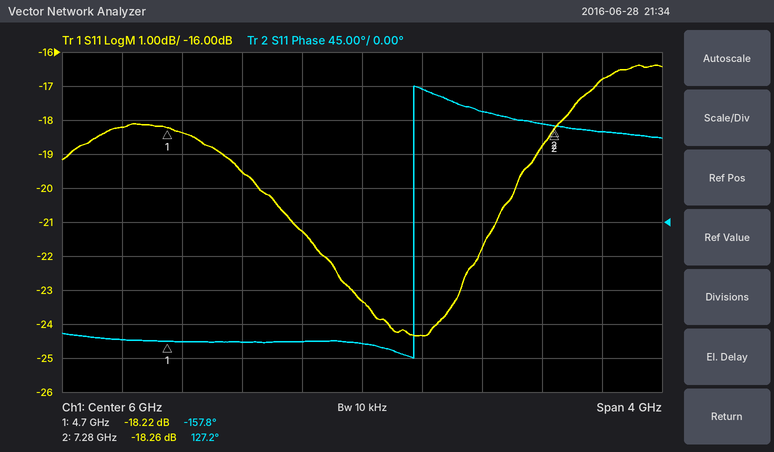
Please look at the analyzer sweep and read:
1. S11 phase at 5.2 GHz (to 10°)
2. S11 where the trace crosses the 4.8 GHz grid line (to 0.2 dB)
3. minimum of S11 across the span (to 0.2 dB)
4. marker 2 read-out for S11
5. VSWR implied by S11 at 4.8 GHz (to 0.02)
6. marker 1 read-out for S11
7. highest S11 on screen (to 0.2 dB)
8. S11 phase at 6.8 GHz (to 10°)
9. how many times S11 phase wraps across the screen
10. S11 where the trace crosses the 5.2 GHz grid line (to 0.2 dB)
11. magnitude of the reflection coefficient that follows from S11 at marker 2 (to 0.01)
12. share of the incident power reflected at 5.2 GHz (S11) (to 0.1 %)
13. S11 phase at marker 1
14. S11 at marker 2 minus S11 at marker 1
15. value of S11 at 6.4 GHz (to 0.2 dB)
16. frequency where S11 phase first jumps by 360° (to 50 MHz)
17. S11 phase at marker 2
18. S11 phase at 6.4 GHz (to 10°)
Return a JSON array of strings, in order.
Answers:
["-160°", "-18.4 dB", "-24.4 dB", "-18.26 dB", "1.28", "-18.22 dB", "-16.4 dB", "150°", "1", "-19.6 dB", "0.12", "1.1 %", "-157.8°", "-0.04 dB", "-24.4 dB", "6.35 GHz", "127.2°", "180°"]
